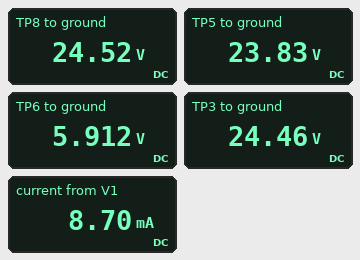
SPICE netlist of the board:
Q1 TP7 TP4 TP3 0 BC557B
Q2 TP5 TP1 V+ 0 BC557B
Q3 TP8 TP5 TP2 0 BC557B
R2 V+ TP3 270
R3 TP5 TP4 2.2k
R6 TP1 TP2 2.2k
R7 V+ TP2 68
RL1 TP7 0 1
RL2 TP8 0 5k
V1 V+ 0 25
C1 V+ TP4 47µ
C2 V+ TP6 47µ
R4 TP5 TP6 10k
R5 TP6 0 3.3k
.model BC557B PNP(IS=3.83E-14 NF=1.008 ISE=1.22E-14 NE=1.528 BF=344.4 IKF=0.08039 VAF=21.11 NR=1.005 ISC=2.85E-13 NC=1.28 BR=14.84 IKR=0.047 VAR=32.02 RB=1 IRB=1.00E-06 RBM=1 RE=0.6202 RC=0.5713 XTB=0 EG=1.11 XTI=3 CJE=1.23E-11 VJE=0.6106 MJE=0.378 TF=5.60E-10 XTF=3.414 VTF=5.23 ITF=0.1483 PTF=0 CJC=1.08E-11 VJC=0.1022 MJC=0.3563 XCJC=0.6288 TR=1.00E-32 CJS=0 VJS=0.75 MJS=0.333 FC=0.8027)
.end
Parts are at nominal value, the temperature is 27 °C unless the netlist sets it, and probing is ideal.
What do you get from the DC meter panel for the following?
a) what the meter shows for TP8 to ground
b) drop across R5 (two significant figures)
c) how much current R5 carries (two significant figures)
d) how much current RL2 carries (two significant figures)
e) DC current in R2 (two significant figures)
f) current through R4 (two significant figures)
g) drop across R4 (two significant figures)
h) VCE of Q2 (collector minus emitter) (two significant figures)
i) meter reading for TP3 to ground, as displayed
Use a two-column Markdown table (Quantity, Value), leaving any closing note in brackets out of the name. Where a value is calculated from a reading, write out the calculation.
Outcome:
| Quantity | Value |
|---|---|
| what the meter shows for TP8 to ground | 24.52 V |
| drop across R5 | 5.912 V = 5.9 V |
| how much current R5 carries | (5.912 V) / 3.3 kΩ = 1.8 mA |
| how much current RL2 carries | (24.52 V) / 5 kΩ = 4.9 mA |
| DC current in R2 | (25 V - 24.46 V) / 270 Ω = 2.0 mA |
| current through R4 | (23.83 V - 5.912 V) / 10 kΩ = 1.8 mA |
| drop across R4 | 23.83 V - 5.912 V = 18 V |
| VCE of Q2 (collector minus emitter) | 23.83 V - 25 V = -1.2 V |
| meter reading for TP3 to ground, as displayed | 24.46 V |
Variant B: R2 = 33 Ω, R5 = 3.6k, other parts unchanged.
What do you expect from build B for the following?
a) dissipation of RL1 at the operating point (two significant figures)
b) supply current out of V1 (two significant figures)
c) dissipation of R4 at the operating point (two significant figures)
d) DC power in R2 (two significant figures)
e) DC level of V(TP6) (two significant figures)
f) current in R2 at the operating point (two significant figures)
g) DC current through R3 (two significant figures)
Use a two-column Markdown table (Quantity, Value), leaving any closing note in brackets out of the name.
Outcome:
| Quantity | Value |
|---|---|
| dissipation of RL1 at the operating point | 180 µW |
| supply current out of V1 | 20 mA |
| dissipation of R4 at the operating point | 31 mW |
| DC power in R2 | 5.9 mW |
| DC level of V(TP6) | 6.3 V |
| current in R2 at the operating point | 13 mA |
| DC current through R3 | 20 µA |
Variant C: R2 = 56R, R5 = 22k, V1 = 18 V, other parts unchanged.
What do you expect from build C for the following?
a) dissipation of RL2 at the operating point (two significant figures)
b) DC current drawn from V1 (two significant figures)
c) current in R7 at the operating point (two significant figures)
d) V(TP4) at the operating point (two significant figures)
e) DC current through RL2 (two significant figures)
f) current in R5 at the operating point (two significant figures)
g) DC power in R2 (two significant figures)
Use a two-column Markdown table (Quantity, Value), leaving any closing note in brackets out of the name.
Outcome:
| Quantity | Value |
|---|---|
| dissipation of RL2 at the operating point | 63 mW |
| DC current drawn from V1 | 9.2 mA |
| current in R7 at the operating point | 4.1 mA |
| V(TP4) at the operating point | 17 V |
| DC current through RL2 | 3.5 mA |
| current in R5 at the operating point | 530 µA |
| DC power in R2 | 1.5 mW |
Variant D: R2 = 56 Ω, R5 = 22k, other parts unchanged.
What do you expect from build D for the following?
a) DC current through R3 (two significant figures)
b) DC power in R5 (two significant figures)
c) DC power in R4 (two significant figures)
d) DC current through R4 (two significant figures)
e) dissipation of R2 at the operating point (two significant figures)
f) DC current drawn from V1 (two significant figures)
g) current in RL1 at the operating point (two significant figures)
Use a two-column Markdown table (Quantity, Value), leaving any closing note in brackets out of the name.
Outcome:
| Quantity | Value |
|---|---|
| DC current through R3 | 10 µA |
| DC power in R5 | 12 mW |
| DC power in R4 | 5.6 mW |
| DC current through R4 | 750 µA |
| dissipation of R2 at the operating point | 2.8 mW |
| DC current drawn from V1 | 13 mA |
| current in RL1 at the operating point | 7.1 mA |
